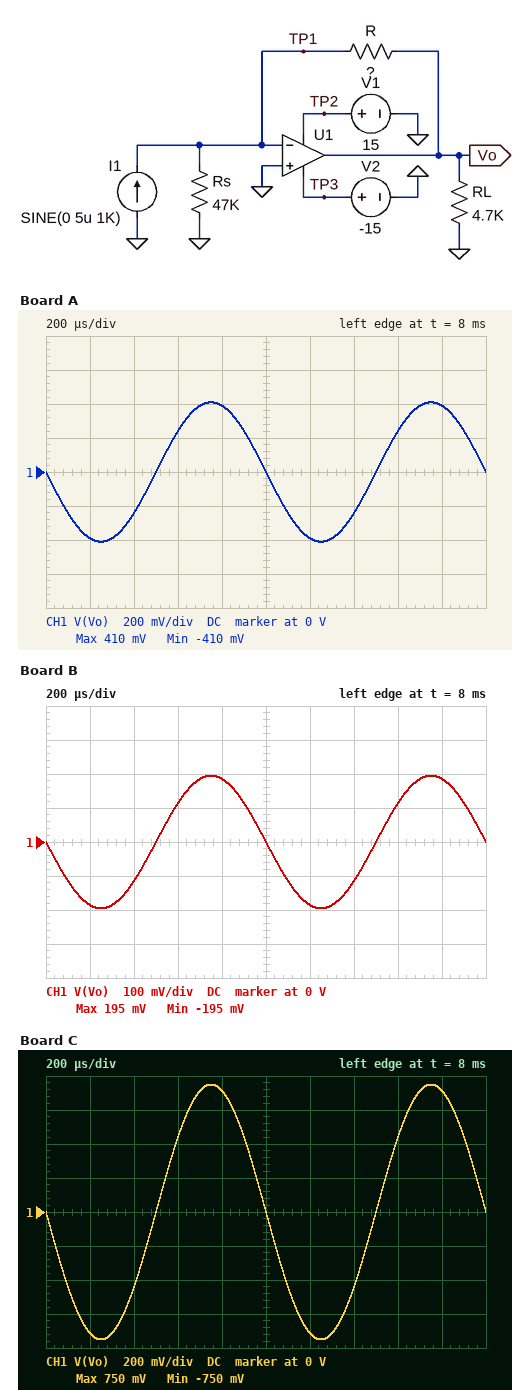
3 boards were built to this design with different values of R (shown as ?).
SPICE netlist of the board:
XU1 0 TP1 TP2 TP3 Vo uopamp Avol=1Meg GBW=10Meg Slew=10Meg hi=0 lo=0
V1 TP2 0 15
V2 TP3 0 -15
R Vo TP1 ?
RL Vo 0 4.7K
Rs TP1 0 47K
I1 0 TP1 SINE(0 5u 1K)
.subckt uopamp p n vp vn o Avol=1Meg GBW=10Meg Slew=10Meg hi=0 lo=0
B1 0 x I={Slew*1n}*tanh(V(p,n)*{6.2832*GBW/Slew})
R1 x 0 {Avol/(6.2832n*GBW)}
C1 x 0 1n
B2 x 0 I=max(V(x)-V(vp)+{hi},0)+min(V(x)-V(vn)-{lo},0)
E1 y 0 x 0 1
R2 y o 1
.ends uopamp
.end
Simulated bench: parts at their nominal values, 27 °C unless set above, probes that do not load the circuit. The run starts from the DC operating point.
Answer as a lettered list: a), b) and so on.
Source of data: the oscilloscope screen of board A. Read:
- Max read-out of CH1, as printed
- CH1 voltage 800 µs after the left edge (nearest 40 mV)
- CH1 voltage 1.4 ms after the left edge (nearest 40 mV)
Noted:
a) 410 mV
b) 400 mV
c) -240 mV
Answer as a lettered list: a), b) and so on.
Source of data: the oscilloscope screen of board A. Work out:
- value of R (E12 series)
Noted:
a) 82 kΩ
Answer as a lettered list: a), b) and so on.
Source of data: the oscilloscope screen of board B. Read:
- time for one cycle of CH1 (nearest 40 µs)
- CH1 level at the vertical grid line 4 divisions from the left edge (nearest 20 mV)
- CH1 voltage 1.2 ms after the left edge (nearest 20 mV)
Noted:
a) 1.00 ms
b) 180 mV
c) -180 mV
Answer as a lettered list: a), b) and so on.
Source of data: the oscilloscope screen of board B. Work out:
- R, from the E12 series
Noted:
a) 39 kΩ
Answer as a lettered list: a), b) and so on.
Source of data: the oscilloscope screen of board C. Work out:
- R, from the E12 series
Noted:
a) 150 kΩ
